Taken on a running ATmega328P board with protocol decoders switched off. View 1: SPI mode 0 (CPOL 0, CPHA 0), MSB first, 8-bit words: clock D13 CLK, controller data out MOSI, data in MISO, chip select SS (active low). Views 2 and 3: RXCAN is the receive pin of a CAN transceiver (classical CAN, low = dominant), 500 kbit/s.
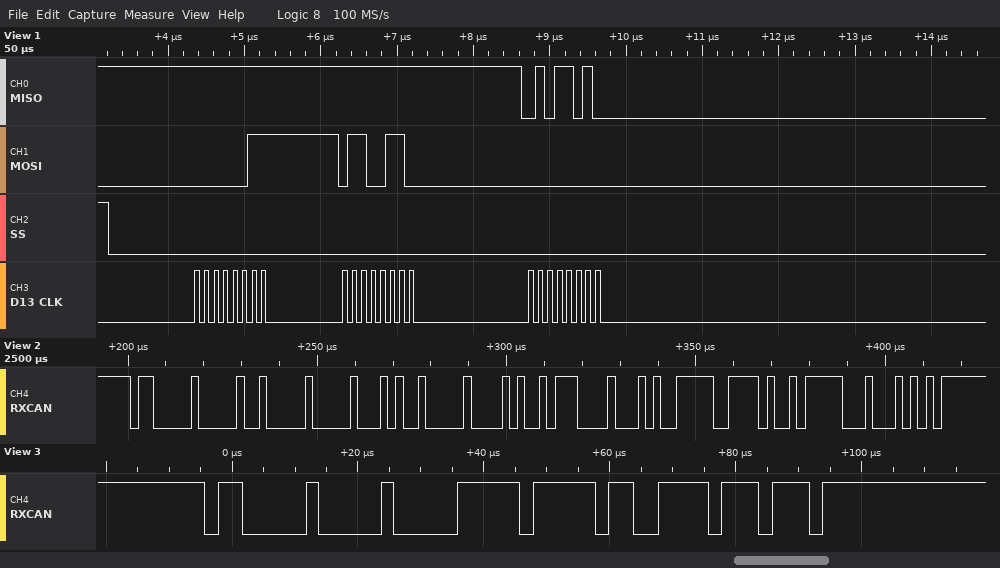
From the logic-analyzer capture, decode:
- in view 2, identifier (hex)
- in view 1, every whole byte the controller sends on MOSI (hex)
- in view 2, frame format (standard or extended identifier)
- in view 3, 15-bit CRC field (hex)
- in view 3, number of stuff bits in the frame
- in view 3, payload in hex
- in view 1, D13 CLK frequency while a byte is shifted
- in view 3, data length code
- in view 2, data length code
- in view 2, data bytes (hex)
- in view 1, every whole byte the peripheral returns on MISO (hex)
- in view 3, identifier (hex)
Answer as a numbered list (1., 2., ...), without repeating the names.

1. 0x600
2. 03 66 00
3. standard
4. 0x67BB
5. 5
6. FF
7. 8 MHz
8. 1
9. 8
10. 00 29 00 52 E1 14 FB D2
11. FF FF 5A
12. 0x600
